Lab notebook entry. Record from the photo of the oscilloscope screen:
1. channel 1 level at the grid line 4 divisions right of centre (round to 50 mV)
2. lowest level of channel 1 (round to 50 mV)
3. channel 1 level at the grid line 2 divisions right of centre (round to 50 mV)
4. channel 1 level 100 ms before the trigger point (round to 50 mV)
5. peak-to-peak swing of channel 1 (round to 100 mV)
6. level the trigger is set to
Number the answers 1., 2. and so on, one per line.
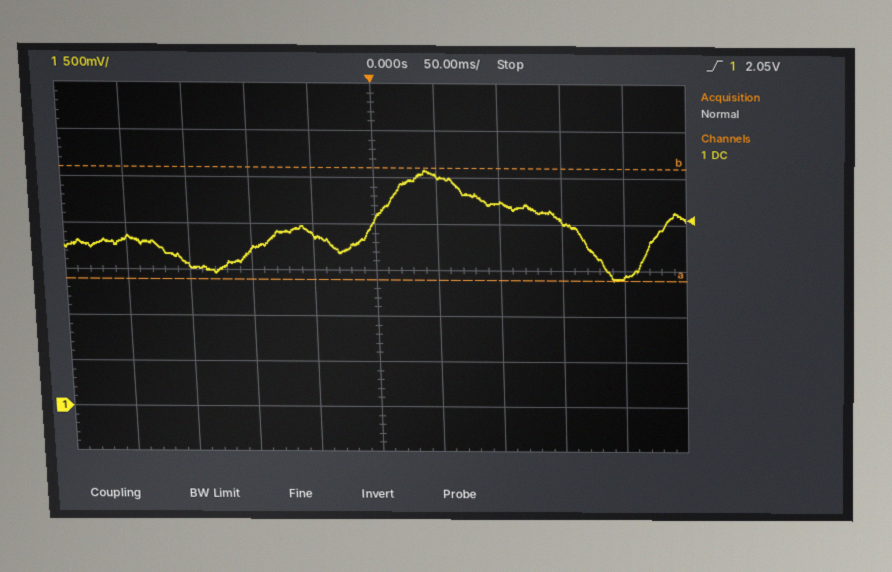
1. 1.45 V
2. 1.40 V
3. 2.25 V
4. 1.70 V
5. 1.20 V
6. 2.05 V
